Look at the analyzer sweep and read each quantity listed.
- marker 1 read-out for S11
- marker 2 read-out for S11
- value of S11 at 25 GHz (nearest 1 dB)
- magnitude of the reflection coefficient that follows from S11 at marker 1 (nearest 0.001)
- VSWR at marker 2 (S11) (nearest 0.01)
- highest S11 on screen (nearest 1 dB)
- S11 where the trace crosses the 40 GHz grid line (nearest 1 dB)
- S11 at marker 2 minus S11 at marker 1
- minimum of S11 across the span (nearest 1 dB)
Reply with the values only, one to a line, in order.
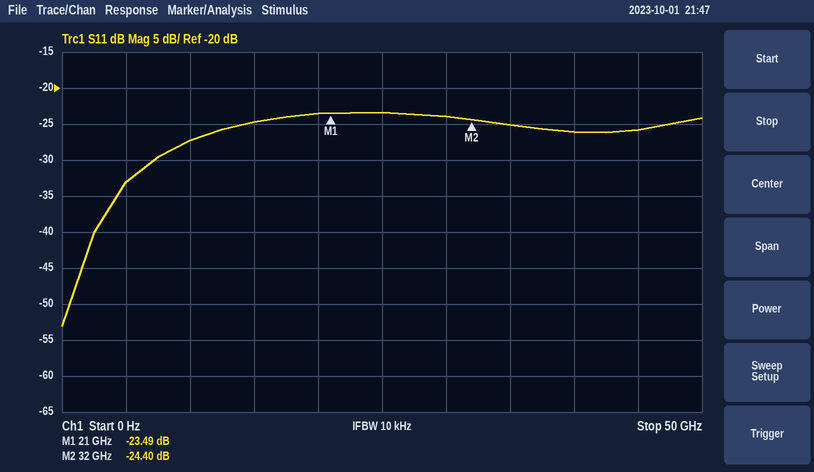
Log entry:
-23.49 dB
-24.40 dB
-23 dB
0.067
1.13
-23 dB
-26 dB
-0.91 dB
-53 dB
